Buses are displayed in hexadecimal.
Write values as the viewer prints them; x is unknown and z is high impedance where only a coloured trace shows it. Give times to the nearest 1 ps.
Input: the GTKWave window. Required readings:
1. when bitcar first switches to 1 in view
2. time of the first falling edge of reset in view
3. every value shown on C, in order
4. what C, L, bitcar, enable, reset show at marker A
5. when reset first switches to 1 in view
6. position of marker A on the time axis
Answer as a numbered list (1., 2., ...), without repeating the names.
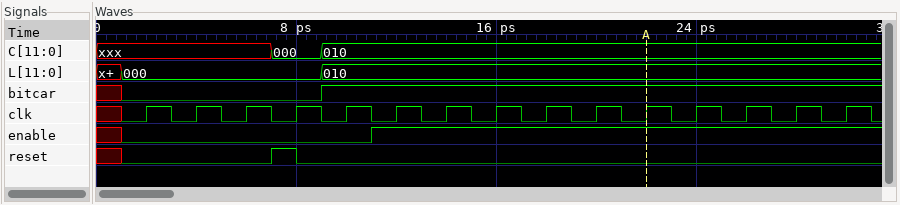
1. 9 ps
2. 8 ps
3. xxx, 000, 010
4. C=010, L=010, bitcar=1, enable=1, reset=0
5. 7 ps
6. 22 ps
